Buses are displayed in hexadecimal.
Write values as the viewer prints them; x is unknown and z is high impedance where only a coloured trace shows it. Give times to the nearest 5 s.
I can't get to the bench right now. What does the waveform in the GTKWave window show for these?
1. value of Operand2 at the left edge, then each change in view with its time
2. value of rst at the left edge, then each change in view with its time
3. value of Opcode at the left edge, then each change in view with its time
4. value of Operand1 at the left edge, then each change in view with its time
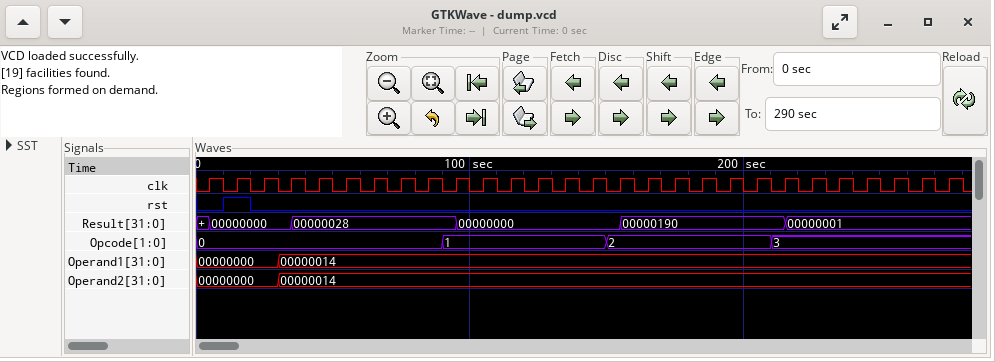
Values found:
00000000, 00000014 at 30 s
0, 1 at 10 s, 0 at 20 s
0, 1 at 90 s, 2 at 150 s, 3 at 210 s
00000000, 00000014 at 30 s
